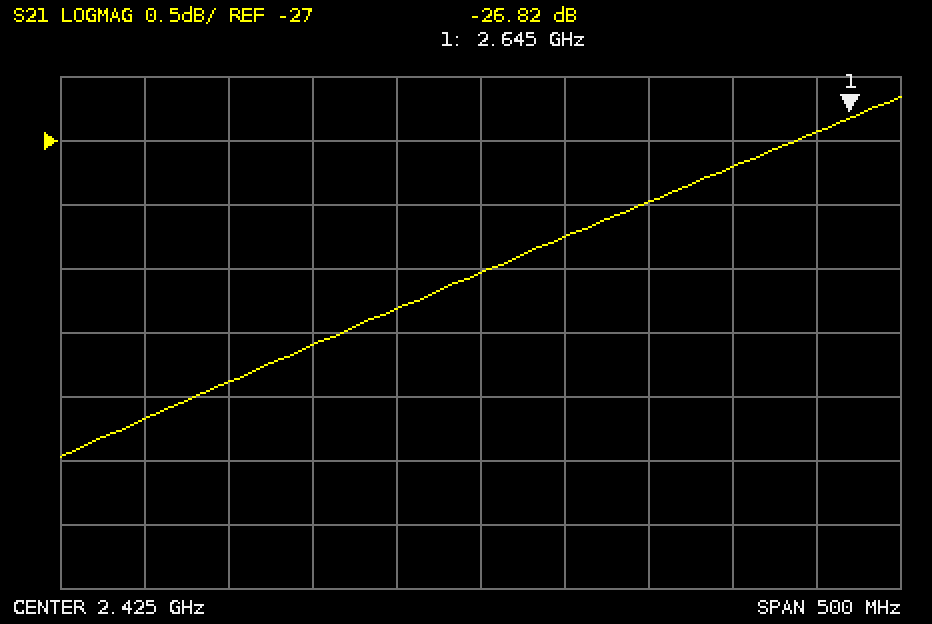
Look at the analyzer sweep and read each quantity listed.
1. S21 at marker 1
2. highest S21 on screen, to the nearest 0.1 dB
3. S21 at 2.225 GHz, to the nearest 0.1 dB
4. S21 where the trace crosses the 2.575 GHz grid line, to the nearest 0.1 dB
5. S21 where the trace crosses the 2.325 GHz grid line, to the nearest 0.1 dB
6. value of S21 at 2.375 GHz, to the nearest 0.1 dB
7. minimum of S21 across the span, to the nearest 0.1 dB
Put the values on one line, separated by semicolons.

-26.82 dB; -26.7 dB; -29.2 dB; -27.2 dB; -28.6 dB; -28.3 dB; -29.5 dB
